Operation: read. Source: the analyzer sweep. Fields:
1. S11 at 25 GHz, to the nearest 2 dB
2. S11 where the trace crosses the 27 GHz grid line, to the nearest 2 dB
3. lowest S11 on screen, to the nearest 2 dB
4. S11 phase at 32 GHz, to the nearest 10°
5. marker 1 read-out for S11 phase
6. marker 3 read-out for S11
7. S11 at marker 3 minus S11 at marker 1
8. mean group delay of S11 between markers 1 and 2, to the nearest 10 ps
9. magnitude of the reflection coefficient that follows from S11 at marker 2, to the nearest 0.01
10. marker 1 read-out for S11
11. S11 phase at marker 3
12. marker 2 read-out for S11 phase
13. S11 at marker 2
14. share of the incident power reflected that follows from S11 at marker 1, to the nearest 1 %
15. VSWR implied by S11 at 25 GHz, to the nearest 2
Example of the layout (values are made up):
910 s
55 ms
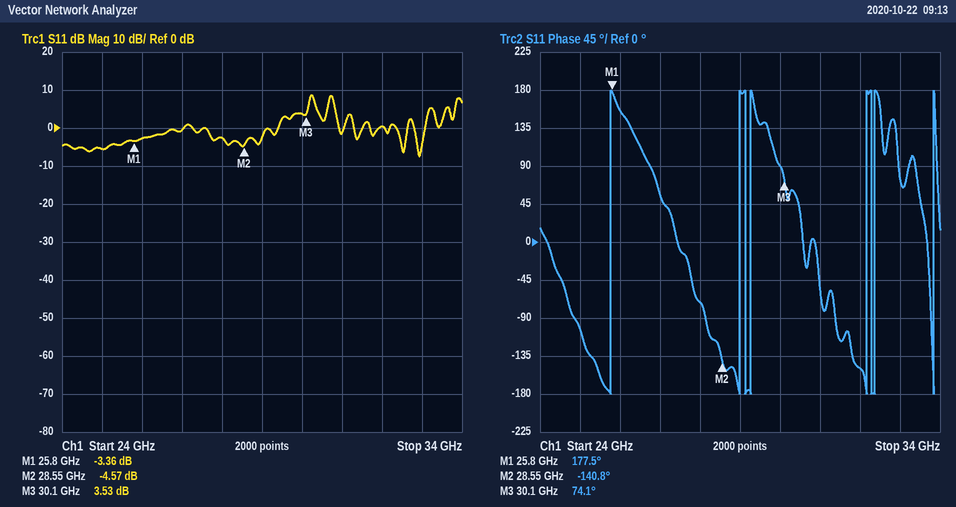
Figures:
-6 dB
0 dB
-8 dB
-150°
177.5°
3.53 dB
6.89 dB
320 ps
0.59
-3.36 dB
74.1°
-140.8°
-4.57 dB
46 %
4
